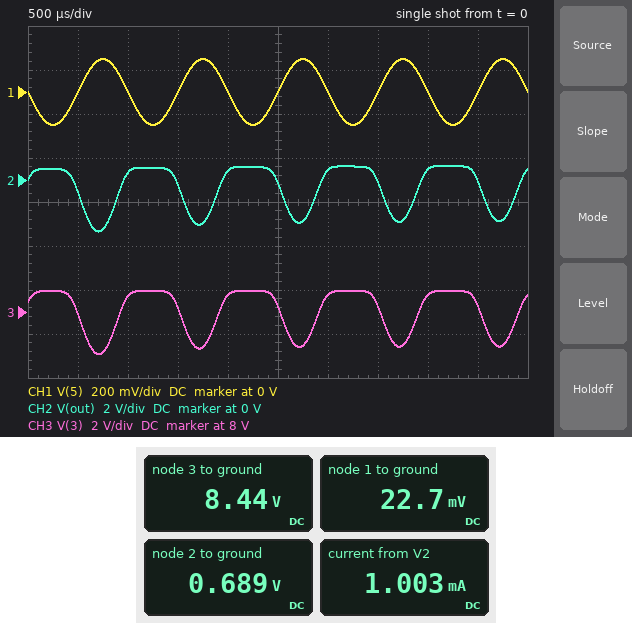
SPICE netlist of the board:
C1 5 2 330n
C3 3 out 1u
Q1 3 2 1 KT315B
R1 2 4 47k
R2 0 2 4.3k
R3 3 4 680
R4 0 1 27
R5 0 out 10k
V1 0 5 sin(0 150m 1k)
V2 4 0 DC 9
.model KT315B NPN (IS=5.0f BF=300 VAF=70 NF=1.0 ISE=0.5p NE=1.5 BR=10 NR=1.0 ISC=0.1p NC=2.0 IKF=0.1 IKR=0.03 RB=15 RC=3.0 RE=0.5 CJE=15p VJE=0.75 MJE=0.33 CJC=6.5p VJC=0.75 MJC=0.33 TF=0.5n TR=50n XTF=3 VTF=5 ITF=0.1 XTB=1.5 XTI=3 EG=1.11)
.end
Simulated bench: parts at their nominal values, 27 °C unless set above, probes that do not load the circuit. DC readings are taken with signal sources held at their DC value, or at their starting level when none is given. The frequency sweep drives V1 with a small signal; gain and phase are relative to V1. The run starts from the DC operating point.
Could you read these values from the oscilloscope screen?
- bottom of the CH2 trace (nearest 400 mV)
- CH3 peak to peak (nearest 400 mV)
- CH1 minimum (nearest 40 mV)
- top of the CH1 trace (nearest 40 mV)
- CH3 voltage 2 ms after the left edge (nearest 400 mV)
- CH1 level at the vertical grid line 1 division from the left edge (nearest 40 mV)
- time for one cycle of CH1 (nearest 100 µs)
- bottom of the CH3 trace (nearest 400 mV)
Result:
-2.4 V
2.8 V
-160 mV
160 mV
8.8 V
0 V
1.0 ms
6.0 V
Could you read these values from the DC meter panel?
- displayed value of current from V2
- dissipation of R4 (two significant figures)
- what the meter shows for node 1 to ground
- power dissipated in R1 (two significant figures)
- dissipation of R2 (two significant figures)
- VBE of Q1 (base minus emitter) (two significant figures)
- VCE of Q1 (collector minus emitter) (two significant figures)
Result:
1.003 mA
19 µW
22.7 mV
1.5 mW
110 µW
670 mV
8.4 V
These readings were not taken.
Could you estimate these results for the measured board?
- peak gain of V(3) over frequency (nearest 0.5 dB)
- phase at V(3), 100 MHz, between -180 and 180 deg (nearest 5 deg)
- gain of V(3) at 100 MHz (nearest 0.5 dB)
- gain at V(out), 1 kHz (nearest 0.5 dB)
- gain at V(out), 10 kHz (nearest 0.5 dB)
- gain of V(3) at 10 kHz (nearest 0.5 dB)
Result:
20.5 dB
-85 deg
14.5 dB
20.5 dB
20.5 dB
20.5 dB
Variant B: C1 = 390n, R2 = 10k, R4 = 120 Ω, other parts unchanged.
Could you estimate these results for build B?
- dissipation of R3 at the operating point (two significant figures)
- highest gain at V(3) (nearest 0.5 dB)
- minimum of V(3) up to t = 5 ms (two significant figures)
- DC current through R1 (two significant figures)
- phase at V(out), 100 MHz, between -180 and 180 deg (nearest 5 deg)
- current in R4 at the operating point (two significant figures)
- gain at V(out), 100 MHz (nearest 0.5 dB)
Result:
9.2 mW
14.0 dB
5.7 V
170 µA
-90 deg
3.7 mA
9.0 dB
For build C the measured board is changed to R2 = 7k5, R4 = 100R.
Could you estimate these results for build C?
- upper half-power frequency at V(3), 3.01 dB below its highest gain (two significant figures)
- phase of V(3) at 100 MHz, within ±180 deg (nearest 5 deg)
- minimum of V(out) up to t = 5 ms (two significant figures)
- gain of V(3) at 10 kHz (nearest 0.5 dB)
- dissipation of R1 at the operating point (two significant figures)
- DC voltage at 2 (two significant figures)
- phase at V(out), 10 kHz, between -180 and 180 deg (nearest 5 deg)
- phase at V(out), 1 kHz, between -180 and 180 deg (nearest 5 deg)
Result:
67 MHz
-90 deg
-930 mV
15.0 dB
1.4 mW
980 mV
0 deg
10 deg
